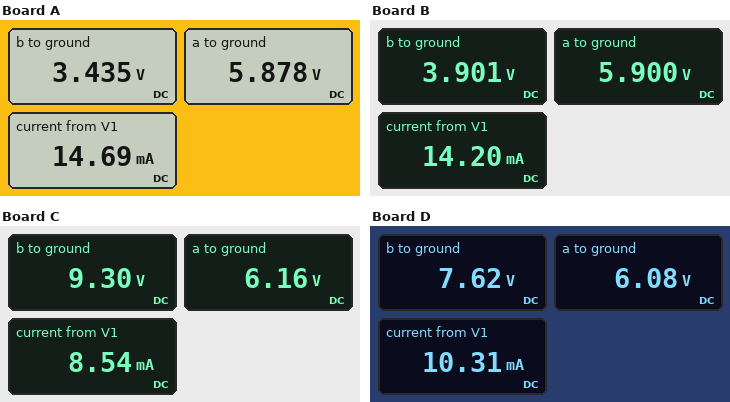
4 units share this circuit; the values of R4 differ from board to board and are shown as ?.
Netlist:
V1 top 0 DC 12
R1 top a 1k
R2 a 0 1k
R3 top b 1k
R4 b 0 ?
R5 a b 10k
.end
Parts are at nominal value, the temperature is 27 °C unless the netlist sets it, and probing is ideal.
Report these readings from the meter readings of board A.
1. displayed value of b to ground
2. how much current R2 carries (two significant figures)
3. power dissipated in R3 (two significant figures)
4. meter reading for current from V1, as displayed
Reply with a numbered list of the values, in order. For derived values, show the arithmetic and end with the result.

1. 3.435 V
2. (5.878 V) / 1 kΩ = 5.9 mA
3. (12 V - 3.435 V)^2 / 1 kΩ = 73 mW
4. 14.69 mA
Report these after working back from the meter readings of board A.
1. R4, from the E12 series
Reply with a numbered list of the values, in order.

1. 390 Ω
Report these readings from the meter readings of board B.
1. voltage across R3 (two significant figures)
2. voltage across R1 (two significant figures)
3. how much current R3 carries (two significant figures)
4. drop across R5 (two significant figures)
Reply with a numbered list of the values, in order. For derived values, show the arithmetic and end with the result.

1. 12 V - 3.901 V = 8.1 V
2. 12 V - 5.9 V = 6.1 V
3. (12 V - 3.901 V) / 1 kΩ = 8.1 mA
4. 5.9 V - 3.901 V = 2.0 V
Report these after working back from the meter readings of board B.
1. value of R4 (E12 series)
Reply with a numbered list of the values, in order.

1. 470 Ω
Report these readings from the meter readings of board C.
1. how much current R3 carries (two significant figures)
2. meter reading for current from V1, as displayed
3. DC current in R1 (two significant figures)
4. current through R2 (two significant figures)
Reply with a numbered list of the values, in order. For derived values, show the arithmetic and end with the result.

1. (12 V - 9.3 V) / 1 kΩ = 2.7 mA
2. 8.54 mA
3. (12 V - 6.16 V) / 1 kΩ = 5.8 mA
4. (6.16 V) / 1 kΩ = 6.2 mA
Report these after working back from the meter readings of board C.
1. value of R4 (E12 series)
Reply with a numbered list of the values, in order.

1. 3.9 kΩ
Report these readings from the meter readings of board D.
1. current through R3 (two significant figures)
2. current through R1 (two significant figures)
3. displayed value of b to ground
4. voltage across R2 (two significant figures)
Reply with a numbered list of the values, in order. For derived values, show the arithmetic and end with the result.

1. (12 V - 7.62 V) / 1 kΩ = 4.4 mA
2. (12 V - 6.08 V) / 1 kΩ = 5.9 mA
3. 7.62 V
4. 6.08 V = 6.1 V
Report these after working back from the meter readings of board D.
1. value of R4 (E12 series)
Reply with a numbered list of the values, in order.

1. 1.8 kΩ
